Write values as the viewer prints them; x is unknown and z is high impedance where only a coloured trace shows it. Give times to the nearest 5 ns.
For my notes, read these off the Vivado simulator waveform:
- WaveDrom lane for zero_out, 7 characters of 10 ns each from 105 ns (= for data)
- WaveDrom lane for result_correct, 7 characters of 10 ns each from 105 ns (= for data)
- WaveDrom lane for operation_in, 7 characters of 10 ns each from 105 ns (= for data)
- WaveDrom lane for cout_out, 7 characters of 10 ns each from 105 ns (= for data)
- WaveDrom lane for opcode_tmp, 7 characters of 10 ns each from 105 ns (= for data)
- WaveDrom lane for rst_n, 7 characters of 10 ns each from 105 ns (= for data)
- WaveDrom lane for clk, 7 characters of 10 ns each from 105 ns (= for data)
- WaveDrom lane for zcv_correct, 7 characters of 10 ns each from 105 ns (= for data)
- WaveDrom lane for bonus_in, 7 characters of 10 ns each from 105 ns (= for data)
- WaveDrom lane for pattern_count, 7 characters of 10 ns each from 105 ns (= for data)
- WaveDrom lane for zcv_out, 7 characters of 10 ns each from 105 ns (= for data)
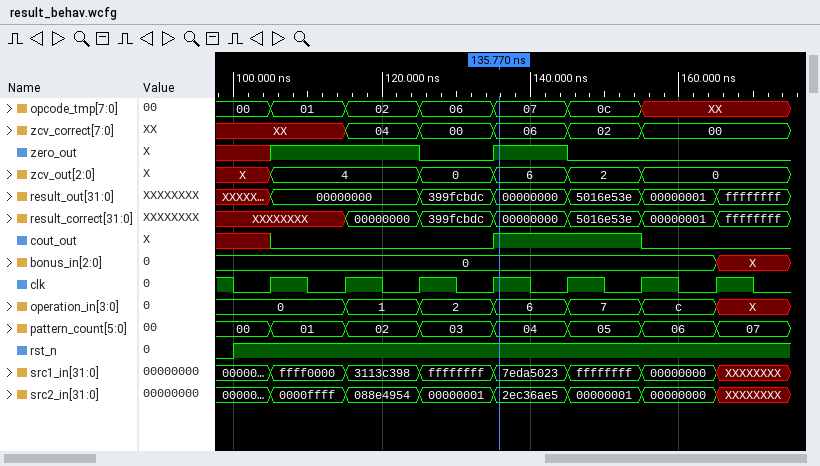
{name: 'zero_out', wave: '1.010..'}
{name: 'result_correct', wave: 'x======', data: '00000000 399fcbdc 00000000 5016e53e 00000001 ffffffff'}
{name: 'operation_in', wave: '======x', data: '0 1 2 6 7 c'}
{name: 'cout_out', wave: '0..1.0.'}
{name: 'opcode_tmp', wave: '=====x.', data: '01 02 06 07 0c'}
{name: 'rst_n', wave: '1......'}
{name: 'clk', wave: 'p......'}
{name: 'zcv_correct', wave: 'x=====.', data: '04 00 06 02 00'}
{name: 'bonus_in', wave: '=.....x', data: '0'}
{name: 'pattern_count', wave: '=======', data: '01 02 03 04 05 06 07'}
{name: 'zcv_out', wave: '=.====.', data: '4 0 6 2 0'}
